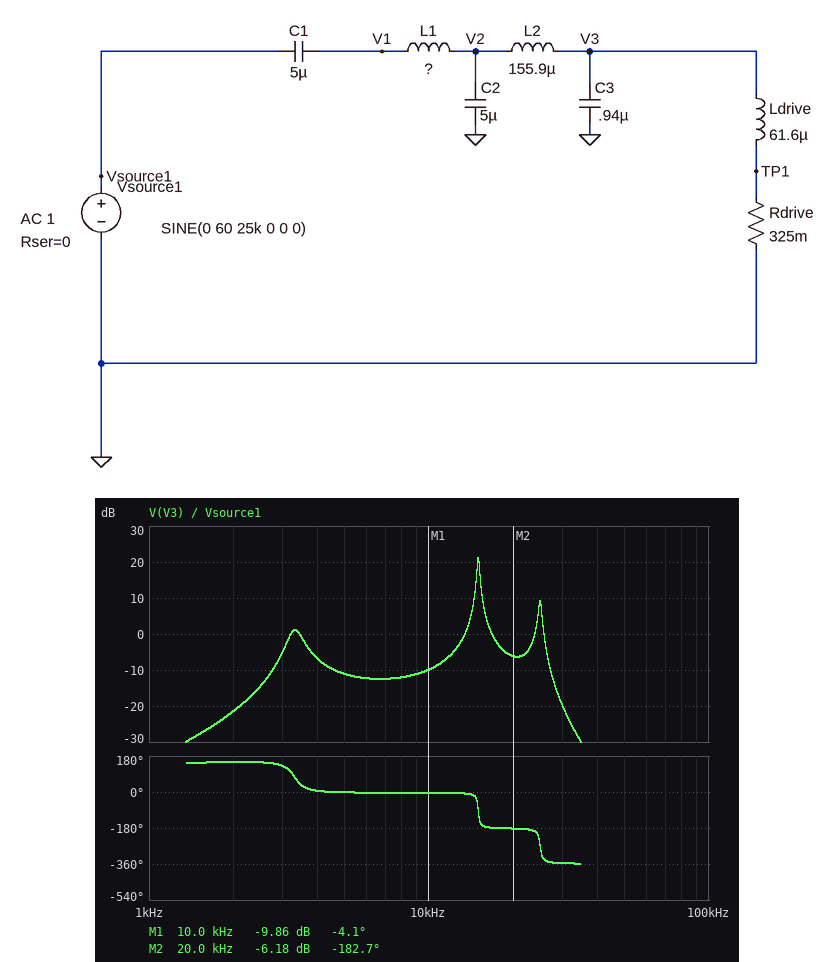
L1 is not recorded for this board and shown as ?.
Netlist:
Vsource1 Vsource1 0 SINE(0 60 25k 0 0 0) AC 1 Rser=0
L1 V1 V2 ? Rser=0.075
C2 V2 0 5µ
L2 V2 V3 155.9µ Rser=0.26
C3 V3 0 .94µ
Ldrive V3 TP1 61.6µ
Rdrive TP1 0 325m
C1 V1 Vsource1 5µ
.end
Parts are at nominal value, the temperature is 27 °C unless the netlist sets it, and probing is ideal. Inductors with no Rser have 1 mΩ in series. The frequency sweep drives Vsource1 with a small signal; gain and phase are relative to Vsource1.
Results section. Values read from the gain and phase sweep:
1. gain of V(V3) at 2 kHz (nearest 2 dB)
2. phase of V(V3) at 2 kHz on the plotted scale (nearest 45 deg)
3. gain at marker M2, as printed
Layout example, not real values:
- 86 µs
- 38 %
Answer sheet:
- -22 dB
- 135 deg
- -6.18 dB
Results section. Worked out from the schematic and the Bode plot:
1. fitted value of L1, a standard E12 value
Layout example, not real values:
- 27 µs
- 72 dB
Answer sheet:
- 47 µH
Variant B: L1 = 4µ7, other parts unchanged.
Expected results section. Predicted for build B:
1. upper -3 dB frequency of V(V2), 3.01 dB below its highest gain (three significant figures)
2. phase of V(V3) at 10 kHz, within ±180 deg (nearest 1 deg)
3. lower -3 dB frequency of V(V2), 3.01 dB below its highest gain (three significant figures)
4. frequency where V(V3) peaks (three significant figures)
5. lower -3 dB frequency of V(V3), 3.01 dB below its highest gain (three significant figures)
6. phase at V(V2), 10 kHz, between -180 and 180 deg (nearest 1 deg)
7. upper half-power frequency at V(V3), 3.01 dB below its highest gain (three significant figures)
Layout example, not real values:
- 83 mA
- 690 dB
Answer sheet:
- 47.8 kHz
- -3 deg
- 45.3 kHz
- 24.8 kHz
- 24.4 kHz
- 0 deg
- 25.1 kHz
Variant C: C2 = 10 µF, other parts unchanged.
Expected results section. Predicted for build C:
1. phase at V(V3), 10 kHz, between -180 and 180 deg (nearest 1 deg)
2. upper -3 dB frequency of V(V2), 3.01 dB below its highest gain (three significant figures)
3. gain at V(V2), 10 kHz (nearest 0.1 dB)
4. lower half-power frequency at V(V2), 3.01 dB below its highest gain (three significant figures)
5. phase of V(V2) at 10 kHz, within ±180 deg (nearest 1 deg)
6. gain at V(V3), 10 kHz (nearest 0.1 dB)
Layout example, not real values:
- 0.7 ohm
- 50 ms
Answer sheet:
- -5 deg
- 13.0 kHz
- -1.1 dB
- 12.7 kHz
- -2 deg
- -10.4 dB
